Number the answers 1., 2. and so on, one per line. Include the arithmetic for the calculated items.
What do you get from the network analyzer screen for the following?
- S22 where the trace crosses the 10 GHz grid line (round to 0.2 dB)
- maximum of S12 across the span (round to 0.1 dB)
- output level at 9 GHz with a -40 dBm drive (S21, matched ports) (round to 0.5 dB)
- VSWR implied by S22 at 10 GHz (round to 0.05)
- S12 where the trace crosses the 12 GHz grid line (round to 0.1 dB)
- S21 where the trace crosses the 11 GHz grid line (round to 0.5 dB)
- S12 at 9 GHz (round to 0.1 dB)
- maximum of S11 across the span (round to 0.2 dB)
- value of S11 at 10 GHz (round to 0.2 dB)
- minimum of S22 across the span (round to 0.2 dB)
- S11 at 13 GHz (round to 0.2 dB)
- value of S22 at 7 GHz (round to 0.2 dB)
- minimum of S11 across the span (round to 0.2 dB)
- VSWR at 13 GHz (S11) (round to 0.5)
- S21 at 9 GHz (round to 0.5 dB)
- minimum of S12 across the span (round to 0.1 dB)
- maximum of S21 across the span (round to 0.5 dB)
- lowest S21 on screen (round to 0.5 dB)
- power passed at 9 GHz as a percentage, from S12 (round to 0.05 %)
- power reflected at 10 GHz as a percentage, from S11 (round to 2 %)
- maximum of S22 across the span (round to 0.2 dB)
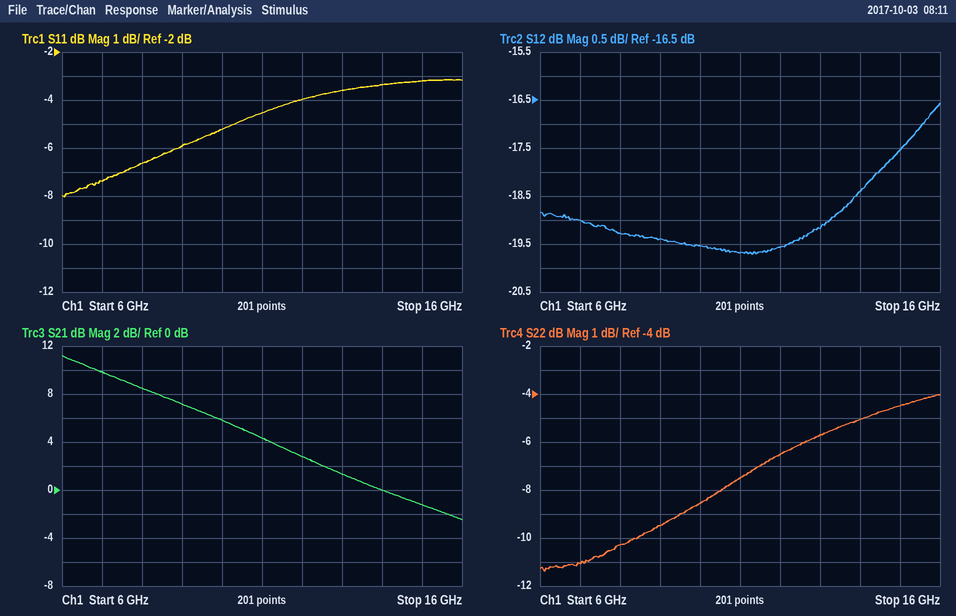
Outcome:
1. -8.6 dB
2. -16.6 dB
3. -40 dBm + (7.0 dB) = -33.0 dBm
4. |Γ| = 10^(-8.6/20) = 0.3715; VSWR = (1 + 0.3715)/(1 − 0.3715) ≈ 2.18, so 2.20 to the nearest 0.05
5. -19.6 dB
6. 4.5 dB
7. -19.4 dB
8. -3.2 dB
9. -5.2 dB
10. -11.4 dB
11. -3.6 dB
12. -11.0 dB
13. -8.0 dB
14. |Γ| = 10^(-3.6/20) = 0.6607; VSWR = (1 + 0.6607)/(1 − 0.6607) ≈ 4.89, so 5.0 to the nearest 0.5
15. 7.0 dB
16. -19.7 dB
17. 11.0 dB
18. -2.5 dB
19. 10^(-19.4/10) ≈ 1.15 %
20. 10^(-5.2/10) ≈ 30 %
21. -4.0 dB
